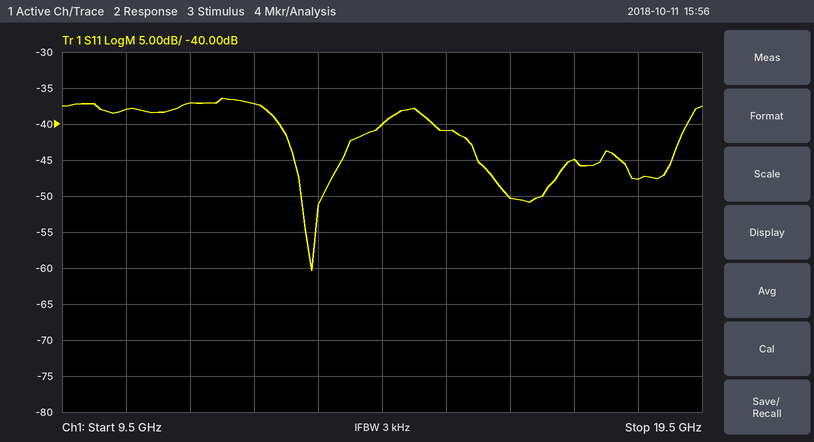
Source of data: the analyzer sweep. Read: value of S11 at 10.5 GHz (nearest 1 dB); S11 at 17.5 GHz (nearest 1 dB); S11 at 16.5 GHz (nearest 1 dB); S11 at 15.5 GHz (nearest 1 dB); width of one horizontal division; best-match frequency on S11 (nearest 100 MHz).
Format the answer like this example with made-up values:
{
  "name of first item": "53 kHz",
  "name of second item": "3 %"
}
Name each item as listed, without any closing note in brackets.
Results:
{
  "value of S11 at 10.5 GHz": "-38 dB",
  "S11 at 17.5 GHz": "-45 dB",
  "S11 at 16.5 GHz": "-50 dB",
  "S11 at 15.5 GHz": "-41 dB",
  "width of one horizontal division": "1 GHz",
  "best-match frequency on S11": "13.4 GHz"
}
